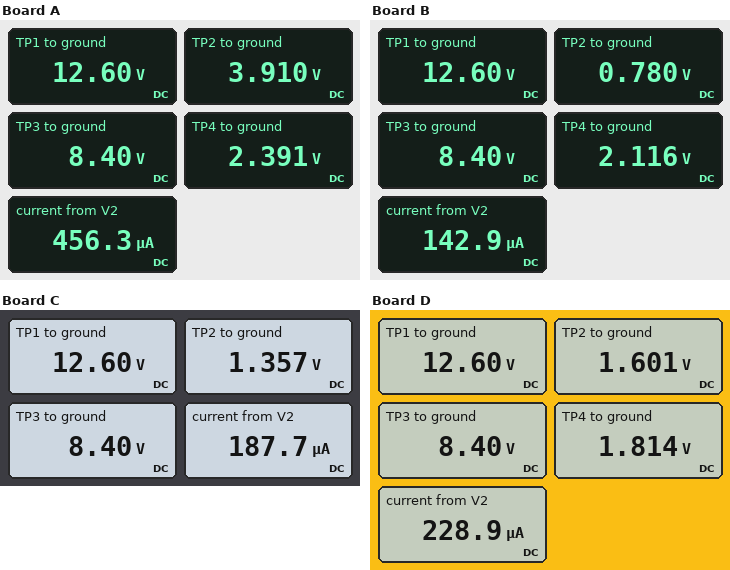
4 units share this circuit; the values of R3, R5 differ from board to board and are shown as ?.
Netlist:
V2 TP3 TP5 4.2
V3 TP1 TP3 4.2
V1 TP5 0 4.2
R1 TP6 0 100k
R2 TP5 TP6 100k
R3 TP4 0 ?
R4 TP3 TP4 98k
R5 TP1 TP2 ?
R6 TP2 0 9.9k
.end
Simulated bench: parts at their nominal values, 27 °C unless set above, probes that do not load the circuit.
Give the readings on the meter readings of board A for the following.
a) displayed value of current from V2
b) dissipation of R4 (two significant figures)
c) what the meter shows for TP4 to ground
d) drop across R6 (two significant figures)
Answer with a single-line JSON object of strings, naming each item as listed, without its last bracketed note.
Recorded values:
{"displayed value of current from V2": "456.3 µA", "dissipation of R4": "370 µW", "what the meter shows for TP4 to ground": "2.391 V", "drop across R6": "3.9 V"}
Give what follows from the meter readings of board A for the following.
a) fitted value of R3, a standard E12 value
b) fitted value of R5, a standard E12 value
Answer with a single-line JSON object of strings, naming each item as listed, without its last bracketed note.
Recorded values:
{"fitted value of R3, a standard E12 value": "39 kΩ", "fitted value of R5, a standard E12 value": "22 kΩ"}
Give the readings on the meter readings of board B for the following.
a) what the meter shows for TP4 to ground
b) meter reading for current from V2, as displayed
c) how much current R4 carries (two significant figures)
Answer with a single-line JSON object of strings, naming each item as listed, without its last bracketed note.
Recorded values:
{"what the meter shows for TP4 to ground": "2.116 V", "meter reading for current from V2, as displayed": "142.9 µA", "how much current R4 carries": "64 µA"}
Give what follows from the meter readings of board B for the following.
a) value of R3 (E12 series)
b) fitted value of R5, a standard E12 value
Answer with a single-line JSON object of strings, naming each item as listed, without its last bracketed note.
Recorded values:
{"value of R3": "33 kΩ", "fitted value of R5, a standard E12 value": "150 kΩ"}
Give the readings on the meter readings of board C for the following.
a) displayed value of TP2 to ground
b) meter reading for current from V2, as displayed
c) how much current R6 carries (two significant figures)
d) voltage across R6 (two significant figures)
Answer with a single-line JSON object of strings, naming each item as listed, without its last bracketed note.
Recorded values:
{"displayed value of TP2 to ground": "1.357 V", "meter reading for current from V2, as displayed": "187.7 µA", "how much current R6 carries": "140 µA", "voltage across R6": "1.4 V"}
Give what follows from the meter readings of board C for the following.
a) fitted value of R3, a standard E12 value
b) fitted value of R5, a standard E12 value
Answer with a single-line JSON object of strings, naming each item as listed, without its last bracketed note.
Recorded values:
{"fitted value of R3, a standard E12 value": "68 kΩ", "fitted value of R5, a standard E12 value": "82 kΩ"}
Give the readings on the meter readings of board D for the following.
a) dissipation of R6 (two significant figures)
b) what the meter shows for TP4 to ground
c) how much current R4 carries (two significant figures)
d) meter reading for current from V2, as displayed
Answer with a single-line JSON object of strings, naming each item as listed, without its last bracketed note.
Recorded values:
{"dissipation of R6": "260 µW", "what the meter shows for TP4 to ground": "1.814 V", "how much current R4 carries": "67 µA", "meter reading for current from V2, as displayed": "228.9 µA"}
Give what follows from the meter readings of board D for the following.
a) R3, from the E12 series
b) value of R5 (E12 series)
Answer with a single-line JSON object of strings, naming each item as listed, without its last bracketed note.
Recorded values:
{"R3, from the E12 series": "27 kΩ", "value of R5": "68 kΩ"}
